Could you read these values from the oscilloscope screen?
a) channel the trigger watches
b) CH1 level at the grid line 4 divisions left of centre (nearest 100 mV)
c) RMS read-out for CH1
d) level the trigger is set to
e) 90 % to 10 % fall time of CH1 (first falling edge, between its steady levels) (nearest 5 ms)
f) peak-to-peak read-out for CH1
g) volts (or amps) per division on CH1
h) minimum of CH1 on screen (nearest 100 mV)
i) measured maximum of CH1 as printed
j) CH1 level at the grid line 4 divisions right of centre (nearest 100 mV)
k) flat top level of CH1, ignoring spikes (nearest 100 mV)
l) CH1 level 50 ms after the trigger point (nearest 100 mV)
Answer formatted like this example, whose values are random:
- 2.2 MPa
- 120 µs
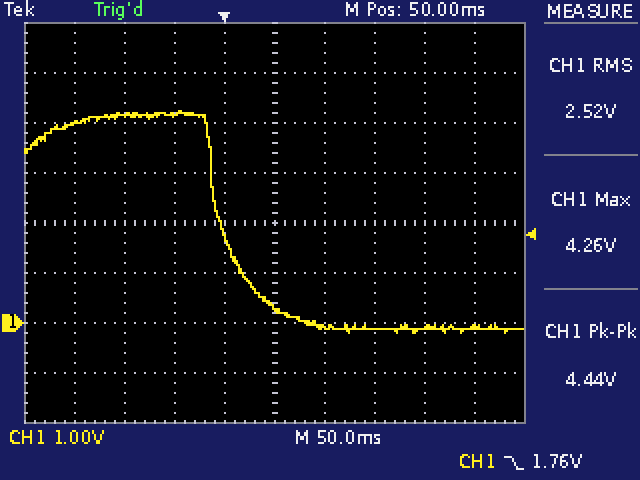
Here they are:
- CH1
- 4.0 V
- 2.52 V
- 1.76 V
- 65 ms
- 4.44 V
- 1 V
- -200 mV
- 4.26 V
- -100 mV
- 4.2 V
- 300 mV
